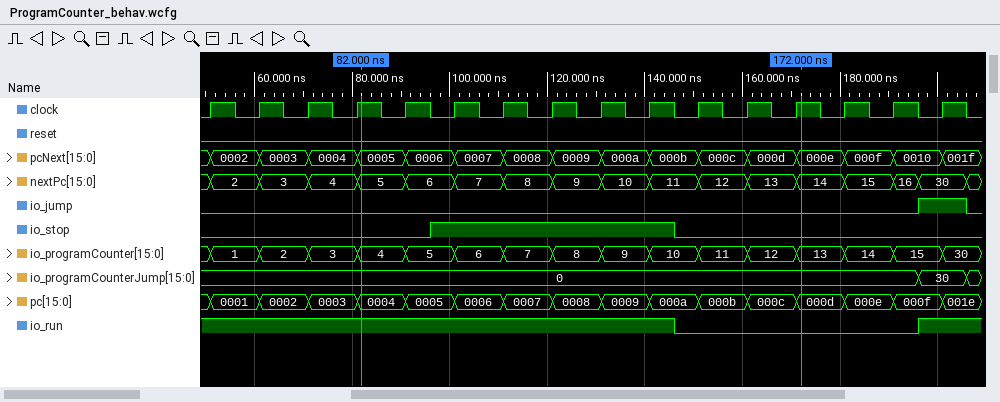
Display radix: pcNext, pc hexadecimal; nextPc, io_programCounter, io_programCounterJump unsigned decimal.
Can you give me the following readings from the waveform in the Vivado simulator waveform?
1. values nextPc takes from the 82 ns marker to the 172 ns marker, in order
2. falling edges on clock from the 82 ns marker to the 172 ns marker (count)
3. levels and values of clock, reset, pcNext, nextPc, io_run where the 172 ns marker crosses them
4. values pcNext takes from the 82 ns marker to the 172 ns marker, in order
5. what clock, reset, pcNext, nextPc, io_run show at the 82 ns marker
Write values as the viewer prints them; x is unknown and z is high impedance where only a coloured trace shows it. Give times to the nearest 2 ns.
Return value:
5, 6, 7, 8, 9, 10, 11, 12, 13, 14
9
clock=1, reset=0, pcNext=000e, nextPc=14, io_run=0
0005, 0006, 0007, 0008, 0009, 000a, 000b, 000c, 000d, 000e
clock=1, reset=0, pcNext=0005, nextPc=5, io_run=1
